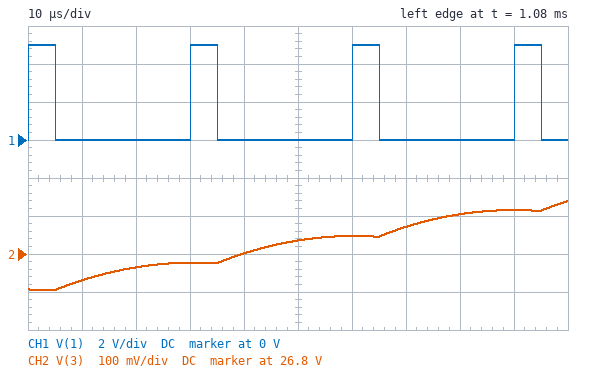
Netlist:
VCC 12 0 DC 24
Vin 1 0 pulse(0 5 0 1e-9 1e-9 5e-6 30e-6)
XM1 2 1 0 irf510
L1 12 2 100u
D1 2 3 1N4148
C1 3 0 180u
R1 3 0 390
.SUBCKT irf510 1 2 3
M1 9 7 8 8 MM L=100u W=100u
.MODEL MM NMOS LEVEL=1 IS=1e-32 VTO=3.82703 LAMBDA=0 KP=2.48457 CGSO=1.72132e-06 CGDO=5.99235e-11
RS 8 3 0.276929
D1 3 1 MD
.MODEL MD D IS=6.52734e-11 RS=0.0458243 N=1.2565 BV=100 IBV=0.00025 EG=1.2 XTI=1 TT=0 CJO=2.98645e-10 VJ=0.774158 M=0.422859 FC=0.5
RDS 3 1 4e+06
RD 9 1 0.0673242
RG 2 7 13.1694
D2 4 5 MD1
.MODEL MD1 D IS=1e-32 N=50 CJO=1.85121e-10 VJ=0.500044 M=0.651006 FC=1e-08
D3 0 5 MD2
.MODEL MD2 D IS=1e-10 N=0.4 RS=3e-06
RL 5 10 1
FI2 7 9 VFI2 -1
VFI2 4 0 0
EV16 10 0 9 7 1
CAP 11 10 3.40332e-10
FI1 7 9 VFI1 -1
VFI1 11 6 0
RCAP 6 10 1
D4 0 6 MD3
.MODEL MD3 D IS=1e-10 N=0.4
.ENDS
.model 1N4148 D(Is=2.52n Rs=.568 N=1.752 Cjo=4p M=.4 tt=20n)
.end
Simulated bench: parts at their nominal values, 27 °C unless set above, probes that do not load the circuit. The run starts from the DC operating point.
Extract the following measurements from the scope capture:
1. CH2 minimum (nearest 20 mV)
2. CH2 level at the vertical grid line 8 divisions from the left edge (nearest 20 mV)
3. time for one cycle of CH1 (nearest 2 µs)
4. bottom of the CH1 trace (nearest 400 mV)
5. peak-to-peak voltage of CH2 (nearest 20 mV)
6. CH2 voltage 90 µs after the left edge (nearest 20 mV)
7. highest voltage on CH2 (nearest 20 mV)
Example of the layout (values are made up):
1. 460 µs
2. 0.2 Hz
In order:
1. 26.70 V
2. 26.90 V
3. 30 µs
4. 0 V
5. 240 mV
6. 26.92 V
7. 26.94 V
